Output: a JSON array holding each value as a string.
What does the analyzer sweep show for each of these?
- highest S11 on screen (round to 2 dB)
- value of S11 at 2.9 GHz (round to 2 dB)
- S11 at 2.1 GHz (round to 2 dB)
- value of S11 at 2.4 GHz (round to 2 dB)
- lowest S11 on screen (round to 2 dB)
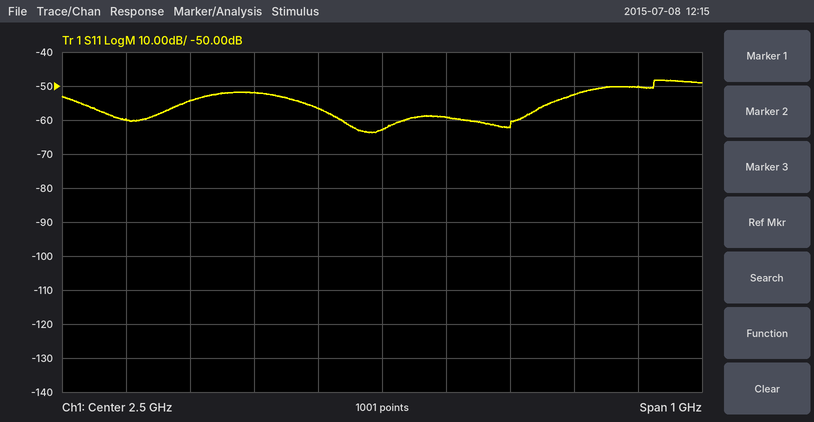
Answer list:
["-48 dB", "-50 dB", "-60 dB", "-56 dB", "-64 dB"]
